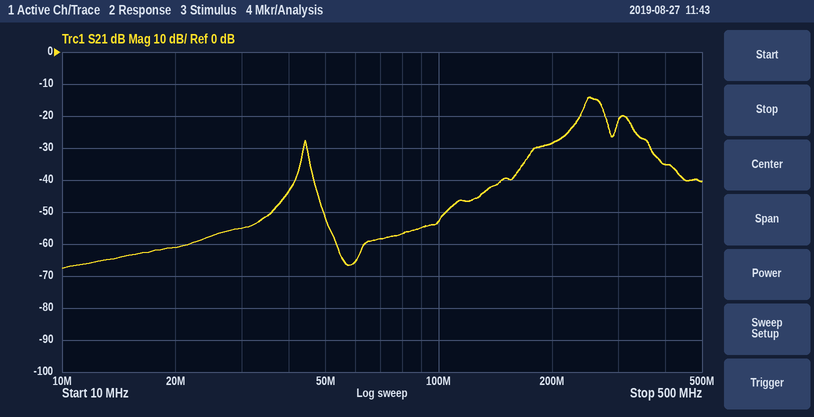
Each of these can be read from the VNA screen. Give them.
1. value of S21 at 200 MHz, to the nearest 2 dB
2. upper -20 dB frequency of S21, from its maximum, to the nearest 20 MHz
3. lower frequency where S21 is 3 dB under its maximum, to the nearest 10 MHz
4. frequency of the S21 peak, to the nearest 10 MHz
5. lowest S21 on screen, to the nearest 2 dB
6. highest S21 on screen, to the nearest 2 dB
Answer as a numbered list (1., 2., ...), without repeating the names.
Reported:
1. -28 dB
2. 380 MHz
3. 240 MHz
4. 250 MHz
5. -68 dB
6. -14 dB
